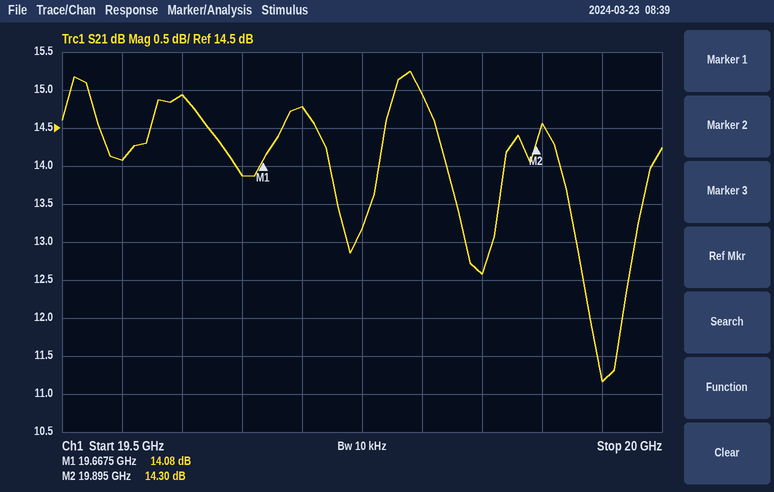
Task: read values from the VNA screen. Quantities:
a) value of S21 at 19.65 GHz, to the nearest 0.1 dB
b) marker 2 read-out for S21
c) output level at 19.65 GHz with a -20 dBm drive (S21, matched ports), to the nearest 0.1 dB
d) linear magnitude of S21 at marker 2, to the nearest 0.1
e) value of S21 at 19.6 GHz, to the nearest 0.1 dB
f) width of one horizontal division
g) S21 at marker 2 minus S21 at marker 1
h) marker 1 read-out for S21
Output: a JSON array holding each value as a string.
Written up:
["13.9 dB", "14.30 dB", "-6.1 dBm", "5.2", "14.9 dB", "50 MHz", "0.22 dB", "14.08 dB"]
